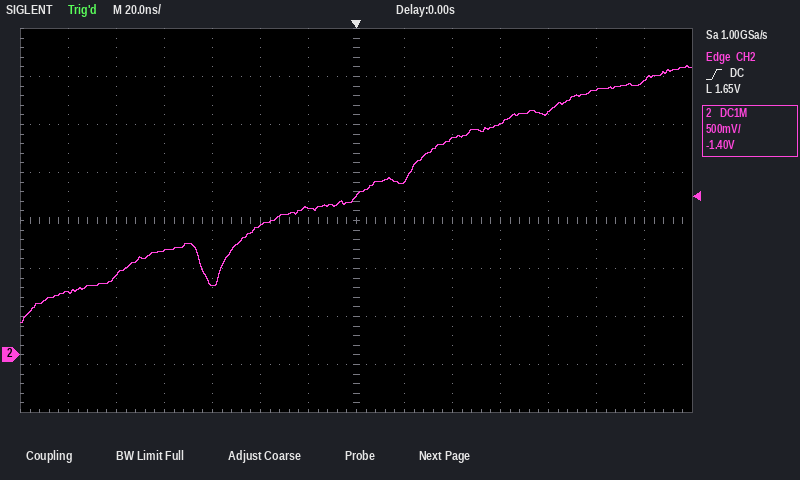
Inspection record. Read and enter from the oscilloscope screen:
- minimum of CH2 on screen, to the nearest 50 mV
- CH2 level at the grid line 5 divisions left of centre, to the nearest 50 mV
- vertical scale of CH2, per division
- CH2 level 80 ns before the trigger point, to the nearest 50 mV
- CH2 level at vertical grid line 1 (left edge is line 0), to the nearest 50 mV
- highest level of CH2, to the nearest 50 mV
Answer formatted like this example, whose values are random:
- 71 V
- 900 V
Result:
- 350 mV
- 850 mV
- 500 mV
- 1.10 V
- 650 mV
- 3.00 V
